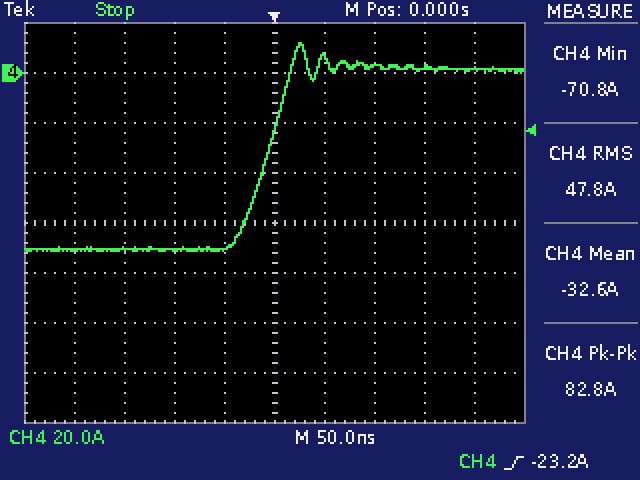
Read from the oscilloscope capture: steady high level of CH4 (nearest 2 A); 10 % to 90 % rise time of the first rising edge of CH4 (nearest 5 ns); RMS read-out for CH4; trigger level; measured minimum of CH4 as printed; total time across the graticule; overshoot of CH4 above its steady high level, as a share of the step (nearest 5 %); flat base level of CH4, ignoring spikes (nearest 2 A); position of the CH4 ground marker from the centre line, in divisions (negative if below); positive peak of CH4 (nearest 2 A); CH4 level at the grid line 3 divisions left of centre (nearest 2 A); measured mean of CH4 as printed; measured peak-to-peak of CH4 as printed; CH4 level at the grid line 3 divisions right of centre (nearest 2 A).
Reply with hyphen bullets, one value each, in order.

- 2 A
- 45 ns
- 47.8 A
- -23.2 A
- -70.8 A
- 500 ns
- 15 %
- -70 A
- +3.0 div
- 12 A
- -70 A
- -32.6 A
- 82.8 A
- 2 A
